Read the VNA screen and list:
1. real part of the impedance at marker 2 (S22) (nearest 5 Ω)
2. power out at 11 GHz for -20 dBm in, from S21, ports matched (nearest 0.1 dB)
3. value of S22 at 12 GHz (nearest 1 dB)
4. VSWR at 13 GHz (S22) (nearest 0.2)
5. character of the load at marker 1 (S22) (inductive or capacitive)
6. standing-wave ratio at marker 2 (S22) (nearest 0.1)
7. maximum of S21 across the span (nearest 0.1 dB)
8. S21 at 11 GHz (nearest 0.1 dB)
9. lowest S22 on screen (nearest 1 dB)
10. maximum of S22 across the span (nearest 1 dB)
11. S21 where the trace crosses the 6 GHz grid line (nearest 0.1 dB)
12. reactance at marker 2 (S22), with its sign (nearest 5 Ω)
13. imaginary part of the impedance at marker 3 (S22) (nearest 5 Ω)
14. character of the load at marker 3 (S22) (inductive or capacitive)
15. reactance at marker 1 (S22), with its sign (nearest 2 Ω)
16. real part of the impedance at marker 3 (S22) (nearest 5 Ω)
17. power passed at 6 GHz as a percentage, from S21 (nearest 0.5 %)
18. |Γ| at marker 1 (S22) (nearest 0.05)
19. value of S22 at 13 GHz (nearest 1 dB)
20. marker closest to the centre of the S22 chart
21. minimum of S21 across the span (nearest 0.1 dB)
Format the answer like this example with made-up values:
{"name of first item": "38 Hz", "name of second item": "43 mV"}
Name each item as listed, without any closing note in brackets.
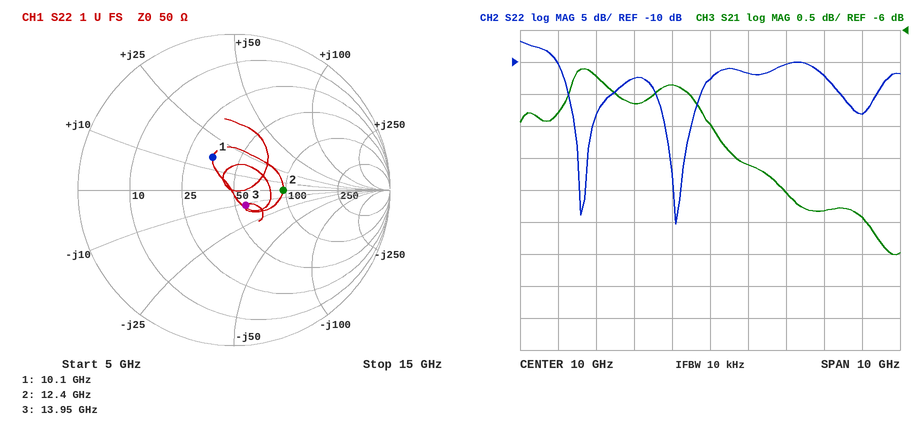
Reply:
{"real part of the impedance at marker 2 (S22)": "95 Ω", "power out at 11 GHz for -20 dBm in, from S21, ports matched": "-28.1 dBm", "value of S22 at 12 GHz": "-10 dB", "VSWR at 13 GHz (S22)": "1.6", "character of the load at marker 1 (S22)": "inductive", "standing-wave ratio at marker 2 (S22)": "1.9", "maximum of S21 across the span": "-6.6 dB", "S21 at 11 GHz": "-8.1 dB", "lowest S22 on screen": "-35 dB", "maximum of S22 across the span": "-7 dB", "S21 where the trace crosses the 6 GHz grid line": "-7.3 dB", "reactance at marker 2 (S22), with its sign": "0 Ω", "imaginary part of the impedance at marker 3 (S22)": "-10 Ω", "character of the load at marker 3 (S22)": "capacitive", "reactance at marker 1 (S22), with its sign": "+16 Ω", "real part of the impedance at marker 3 (S22)": "55 Ω", "power passed at 6 GHz as a percentage, from S21": "18.5 %", "|Γ| at marker 1 (S22)": "0.25", "value of S22 at 13 GHz": "-12 dB", "marker closest to the centre of the S22 chart": "marker 3", "minimum of S21 across the span": "-9.5 dB"}
